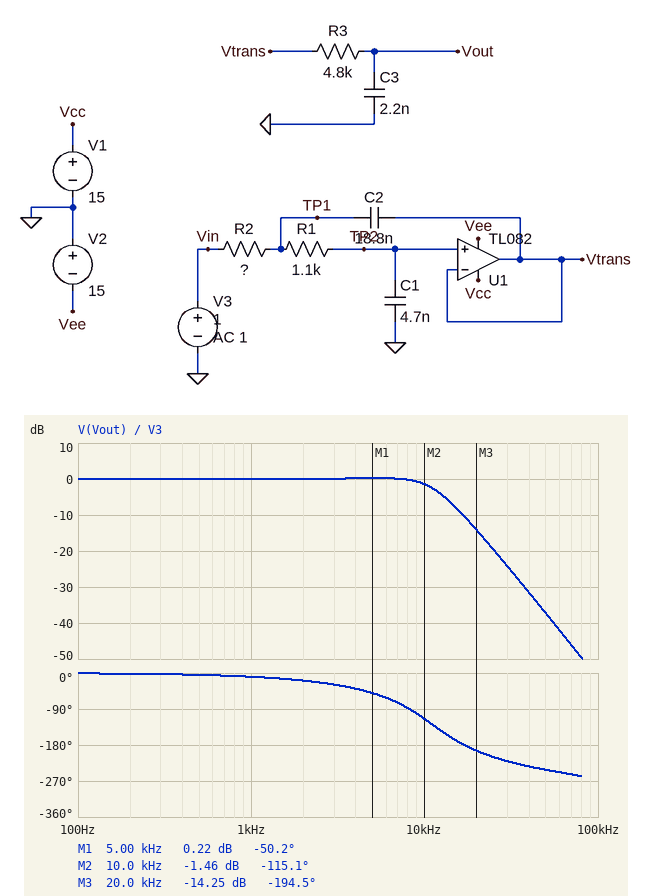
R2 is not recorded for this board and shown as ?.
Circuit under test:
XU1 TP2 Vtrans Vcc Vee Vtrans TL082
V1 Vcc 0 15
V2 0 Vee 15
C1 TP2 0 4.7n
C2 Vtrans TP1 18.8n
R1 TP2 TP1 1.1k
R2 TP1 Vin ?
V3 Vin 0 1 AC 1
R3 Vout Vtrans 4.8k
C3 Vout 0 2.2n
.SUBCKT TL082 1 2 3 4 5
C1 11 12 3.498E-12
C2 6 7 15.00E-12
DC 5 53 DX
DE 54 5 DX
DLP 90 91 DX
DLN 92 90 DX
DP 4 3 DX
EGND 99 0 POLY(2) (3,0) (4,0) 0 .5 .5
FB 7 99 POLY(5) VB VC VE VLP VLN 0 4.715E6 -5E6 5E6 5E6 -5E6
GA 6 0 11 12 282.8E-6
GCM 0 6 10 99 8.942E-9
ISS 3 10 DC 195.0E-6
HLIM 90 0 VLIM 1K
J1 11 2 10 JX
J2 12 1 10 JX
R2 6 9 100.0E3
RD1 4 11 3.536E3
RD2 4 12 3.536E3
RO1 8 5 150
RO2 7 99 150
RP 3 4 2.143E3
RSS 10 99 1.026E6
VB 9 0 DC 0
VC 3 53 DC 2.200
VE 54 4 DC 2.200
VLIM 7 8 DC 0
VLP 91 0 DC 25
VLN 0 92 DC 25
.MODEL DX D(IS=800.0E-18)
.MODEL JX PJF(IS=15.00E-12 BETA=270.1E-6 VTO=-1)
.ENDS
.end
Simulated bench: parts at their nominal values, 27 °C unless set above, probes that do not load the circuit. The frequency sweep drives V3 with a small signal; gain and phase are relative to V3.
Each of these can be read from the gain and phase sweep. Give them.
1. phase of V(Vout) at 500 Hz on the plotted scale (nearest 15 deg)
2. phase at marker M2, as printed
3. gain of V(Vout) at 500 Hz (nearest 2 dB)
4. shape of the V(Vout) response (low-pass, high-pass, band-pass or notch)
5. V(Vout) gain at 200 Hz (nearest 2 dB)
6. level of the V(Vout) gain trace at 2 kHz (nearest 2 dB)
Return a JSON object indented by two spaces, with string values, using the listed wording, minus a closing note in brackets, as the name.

{
  "phase of V(Vout) at 500 Hz on the plotted scale": "0 deg",
  "phase at marker M2, as printed": "-115.1 deg",
  "gain of V(Vout) at 500 Hz": "0 dB",
  "shape of the V(Vout) response": "low-pass",
  "V(Vout) gain at 200 Hz": "0 dB",
  "level of the V(Vout) gain trace at 2 kHz": "0 dB"
}
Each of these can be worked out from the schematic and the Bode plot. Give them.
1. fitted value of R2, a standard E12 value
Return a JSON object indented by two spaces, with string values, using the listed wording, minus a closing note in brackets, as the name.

{
  "fitted value of R2, a standard E12 value": "2.2 kΩ"
}
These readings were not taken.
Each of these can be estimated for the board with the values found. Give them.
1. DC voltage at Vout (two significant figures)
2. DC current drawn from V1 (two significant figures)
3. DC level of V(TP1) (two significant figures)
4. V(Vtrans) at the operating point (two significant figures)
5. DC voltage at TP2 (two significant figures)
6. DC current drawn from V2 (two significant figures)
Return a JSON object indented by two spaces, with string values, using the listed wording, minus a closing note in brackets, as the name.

{
  "DC voltage at Vout": "1.0 V",
  "DC current drawn from V1": "14 mA",
  "DC level of V(TP1)": "1.0 V",
  "V(Vtrans) at the operating point": "1.0 V",
  "DC voltage at TP2": "1.0 V",
  "DC current drawn from V2": "14 mA"
}
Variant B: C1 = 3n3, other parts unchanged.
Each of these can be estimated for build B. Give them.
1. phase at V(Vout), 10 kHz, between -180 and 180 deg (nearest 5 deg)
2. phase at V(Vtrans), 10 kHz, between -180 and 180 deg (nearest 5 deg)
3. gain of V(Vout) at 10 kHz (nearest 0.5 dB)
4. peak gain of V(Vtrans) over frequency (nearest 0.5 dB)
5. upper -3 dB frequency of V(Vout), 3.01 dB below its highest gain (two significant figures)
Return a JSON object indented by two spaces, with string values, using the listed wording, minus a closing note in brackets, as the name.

{
  "phase at V(Vout), 10 kHz, between -180 and 180 deg": "-95 deg",
  "phase at V(Vtrans), 10 kHz, between -180 and 180 deg": "-60 deg",
  "gain of V(Vout) at 10 kHz": "0.5 dB",
  "peak gain of V(Vtrans) over frequency": "2.0 dB",
  "upper -3 dB frequency of V(Vout), 3.01 dB below its highest gain": "14 kHz"
}
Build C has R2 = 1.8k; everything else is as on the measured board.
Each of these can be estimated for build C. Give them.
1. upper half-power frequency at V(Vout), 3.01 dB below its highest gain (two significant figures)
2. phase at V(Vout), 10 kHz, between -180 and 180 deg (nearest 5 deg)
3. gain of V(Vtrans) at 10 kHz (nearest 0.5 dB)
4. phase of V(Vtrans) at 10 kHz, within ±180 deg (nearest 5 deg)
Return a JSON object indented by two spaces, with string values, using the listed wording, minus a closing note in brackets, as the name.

{
  "upper half-power frequency at V(Vout), 3.01 dB below its highest gain": "12 kHz",
  "phase at V(Vout), 10 kHz, between -180 and 180 deg": "-105 deg",
  "gain of V(Vtrans) at 10 kHz": "1.0 dB",
  "phase of V(Vtrans) at 10 kHz, within ±180 deg": "-70 deg"
}
